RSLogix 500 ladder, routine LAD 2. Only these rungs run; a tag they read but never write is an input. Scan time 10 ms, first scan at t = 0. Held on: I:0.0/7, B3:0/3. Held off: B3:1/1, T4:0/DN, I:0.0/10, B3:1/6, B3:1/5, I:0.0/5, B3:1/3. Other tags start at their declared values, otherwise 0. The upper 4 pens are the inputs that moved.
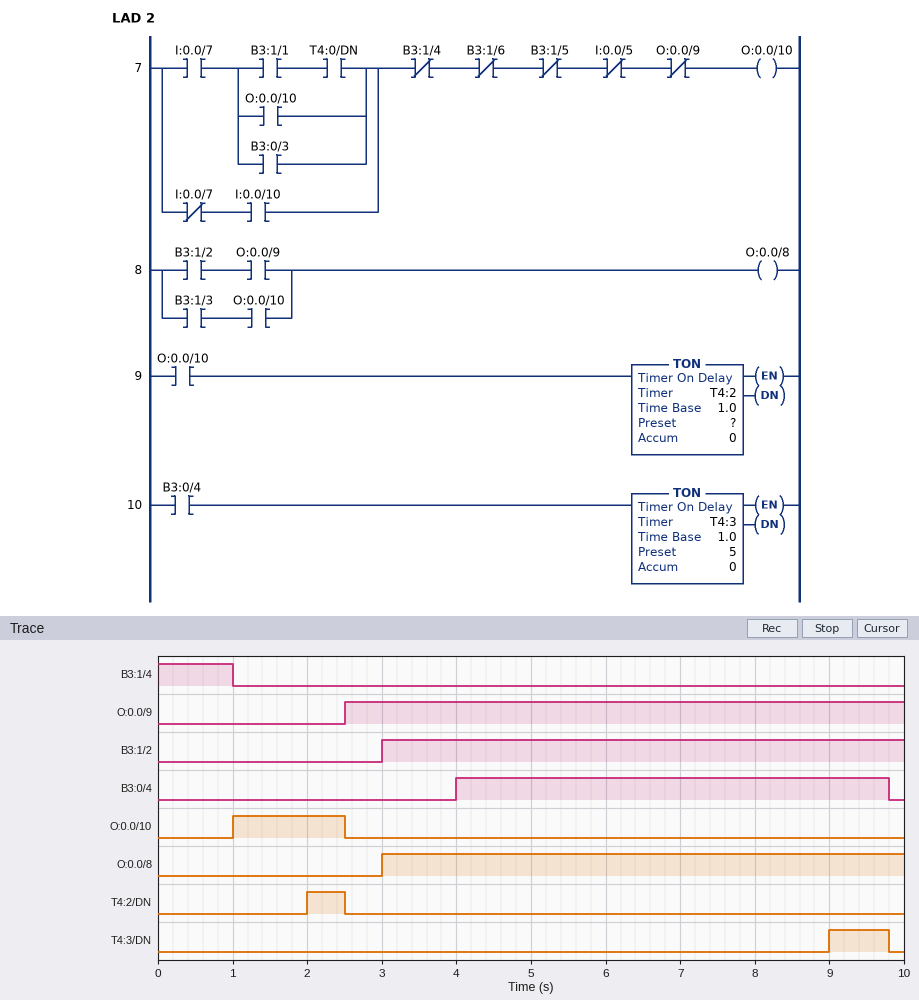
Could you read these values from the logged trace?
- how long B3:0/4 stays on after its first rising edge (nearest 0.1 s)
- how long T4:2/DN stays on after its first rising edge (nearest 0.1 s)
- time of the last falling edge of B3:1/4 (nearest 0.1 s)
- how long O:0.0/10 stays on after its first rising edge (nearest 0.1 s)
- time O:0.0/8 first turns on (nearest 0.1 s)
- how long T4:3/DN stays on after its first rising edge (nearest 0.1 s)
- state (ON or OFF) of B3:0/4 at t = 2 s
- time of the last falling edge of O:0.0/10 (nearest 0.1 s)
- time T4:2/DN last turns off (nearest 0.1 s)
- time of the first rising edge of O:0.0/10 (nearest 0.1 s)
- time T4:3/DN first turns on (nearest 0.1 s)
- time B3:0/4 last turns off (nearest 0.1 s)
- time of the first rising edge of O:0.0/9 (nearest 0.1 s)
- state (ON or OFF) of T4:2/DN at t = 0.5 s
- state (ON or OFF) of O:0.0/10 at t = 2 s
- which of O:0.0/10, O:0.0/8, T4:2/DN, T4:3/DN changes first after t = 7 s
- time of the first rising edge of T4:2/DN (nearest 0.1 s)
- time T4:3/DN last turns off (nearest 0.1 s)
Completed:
5.8 s
0.5 s
1.0 s
1.5 s
3.0 s
0.8 s
OFF
2.5 s
2.5 s
1.0 s
9.0 s
9.8 s
2.5 s
OFF
ON
T4:3/DN
2.0 s
9.8 s
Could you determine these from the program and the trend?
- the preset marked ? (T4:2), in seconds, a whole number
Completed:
1 s
